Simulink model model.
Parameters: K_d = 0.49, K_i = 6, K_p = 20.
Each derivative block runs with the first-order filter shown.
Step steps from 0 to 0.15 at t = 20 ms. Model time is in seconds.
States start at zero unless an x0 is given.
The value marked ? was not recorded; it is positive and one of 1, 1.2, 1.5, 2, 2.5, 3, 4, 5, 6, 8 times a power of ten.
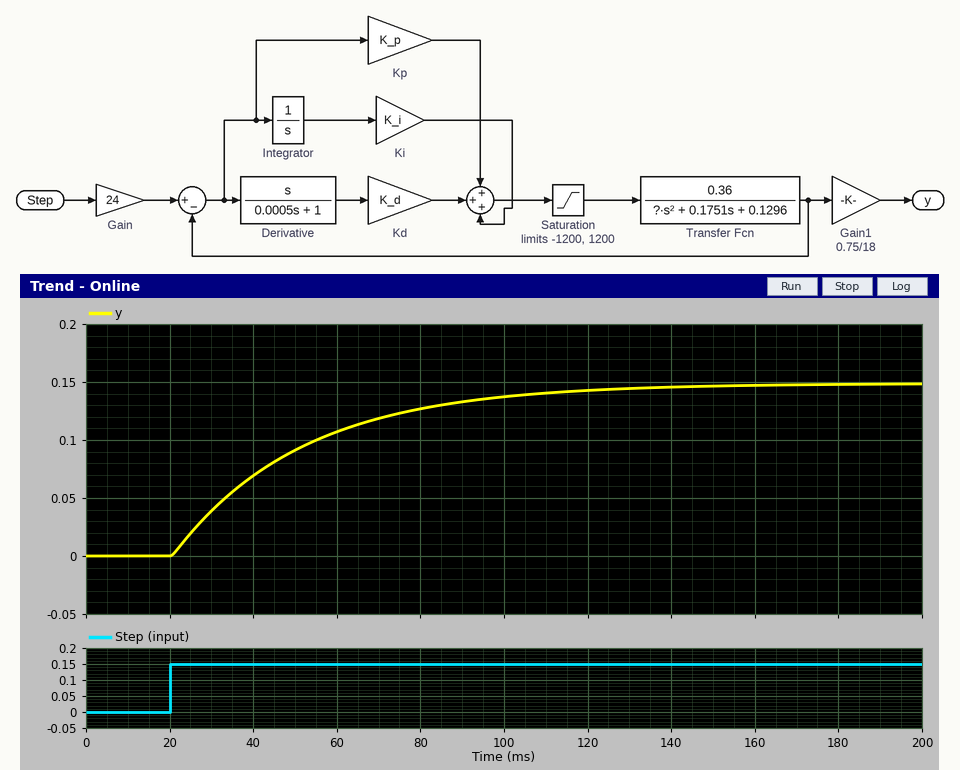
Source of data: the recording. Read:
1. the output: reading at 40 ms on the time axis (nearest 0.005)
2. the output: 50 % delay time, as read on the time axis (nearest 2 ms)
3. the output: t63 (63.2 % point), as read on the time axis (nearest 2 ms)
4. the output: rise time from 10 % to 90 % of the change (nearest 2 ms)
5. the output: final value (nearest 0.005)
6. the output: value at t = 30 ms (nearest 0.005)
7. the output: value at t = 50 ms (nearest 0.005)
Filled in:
0.070
42 ms
52 ms
68 ms
0.150
0.040
0.090
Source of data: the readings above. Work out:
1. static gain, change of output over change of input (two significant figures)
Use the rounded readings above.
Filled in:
1.0
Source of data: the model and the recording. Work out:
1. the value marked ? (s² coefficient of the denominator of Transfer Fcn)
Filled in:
0.004
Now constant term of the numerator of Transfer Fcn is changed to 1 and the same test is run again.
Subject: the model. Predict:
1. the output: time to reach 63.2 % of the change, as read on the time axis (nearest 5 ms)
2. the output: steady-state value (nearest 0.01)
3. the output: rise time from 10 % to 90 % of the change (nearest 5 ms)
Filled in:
35 ms
0.15
40 ms
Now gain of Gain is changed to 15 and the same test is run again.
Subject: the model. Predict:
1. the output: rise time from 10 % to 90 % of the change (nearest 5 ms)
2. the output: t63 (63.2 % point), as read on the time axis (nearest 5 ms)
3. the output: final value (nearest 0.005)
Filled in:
60 ms
45 ms
0.095
